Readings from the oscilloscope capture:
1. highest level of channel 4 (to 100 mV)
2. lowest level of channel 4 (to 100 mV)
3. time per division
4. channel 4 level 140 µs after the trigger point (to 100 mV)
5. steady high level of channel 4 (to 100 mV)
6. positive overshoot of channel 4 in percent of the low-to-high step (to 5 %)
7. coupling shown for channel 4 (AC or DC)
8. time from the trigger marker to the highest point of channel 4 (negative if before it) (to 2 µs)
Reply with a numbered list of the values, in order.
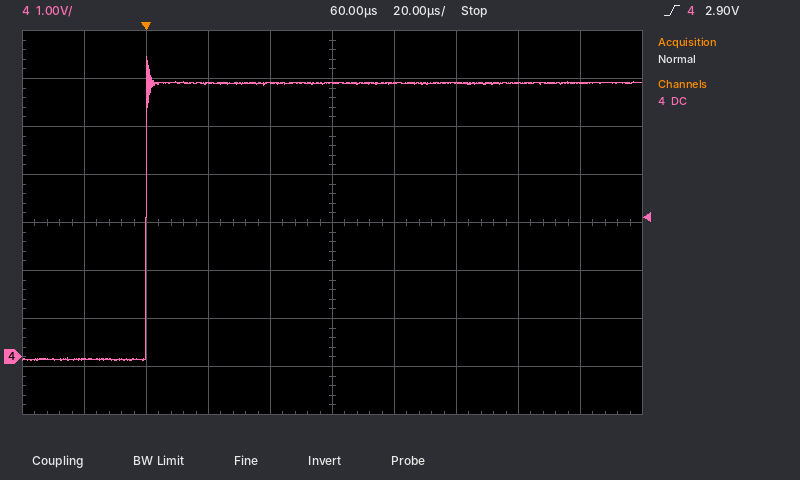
1. 6.3 V
2. -100 mV
3. 20 µs
4. 5.7 V
5. 5.7 V
6. 10 %
7. DC
8. 0 µs
